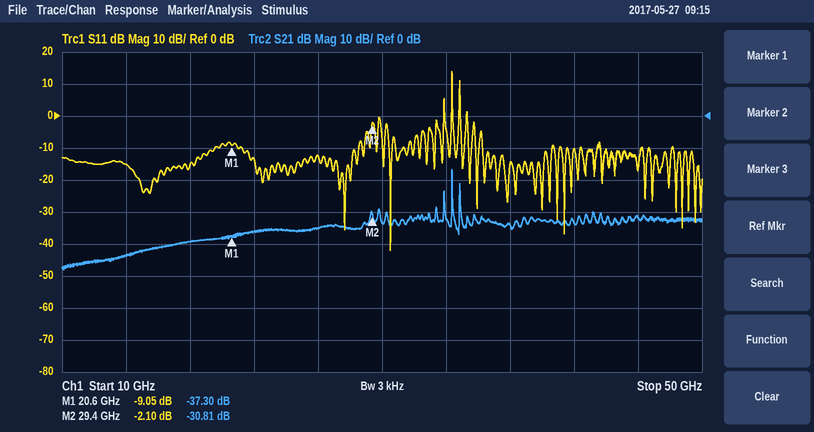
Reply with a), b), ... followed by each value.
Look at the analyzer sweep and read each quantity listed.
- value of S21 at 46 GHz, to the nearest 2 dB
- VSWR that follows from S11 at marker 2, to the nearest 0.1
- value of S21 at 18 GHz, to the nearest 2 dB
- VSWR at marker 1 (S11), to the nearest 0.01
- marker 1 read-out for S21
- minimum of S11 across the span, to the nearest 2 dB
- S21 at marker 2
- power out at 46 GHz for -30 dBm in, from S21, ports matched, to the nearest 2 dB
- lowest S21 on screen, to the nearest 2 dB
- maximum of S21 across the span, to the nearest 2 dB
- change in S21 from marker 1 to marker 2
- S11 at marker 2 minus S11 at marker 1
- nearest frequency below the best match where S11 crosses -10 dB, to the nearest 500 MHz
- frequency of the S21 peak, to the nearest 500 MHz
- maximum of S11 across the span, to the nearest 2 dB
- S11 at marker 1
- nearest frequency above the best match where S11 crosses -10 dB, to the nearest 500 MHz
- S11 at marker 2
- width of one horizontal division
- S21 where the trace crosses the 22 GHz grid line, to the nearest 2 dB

a) -32 dB
b) 8.3
c) -40 dB
d) 2.09
e) -37.30 dB
f) -42 dB
g) -30.81 dB
h) -62 dBm
i) -48 dB
j) -16 dB
k) 6.49 dB
l) 6.95 dB
m) 30.5 GHz
n) 34.5 GHz
o) 14 dB
p) -9.05 dB
q) 30.5 GHz
r) -2.10 dB
s) 4 GHz
t) -36 dB
